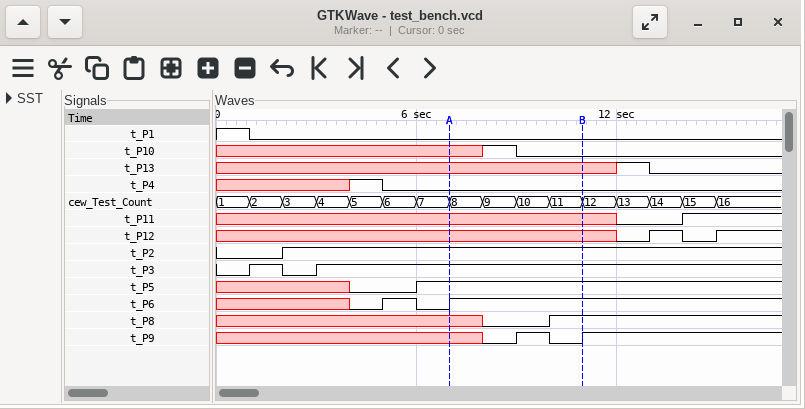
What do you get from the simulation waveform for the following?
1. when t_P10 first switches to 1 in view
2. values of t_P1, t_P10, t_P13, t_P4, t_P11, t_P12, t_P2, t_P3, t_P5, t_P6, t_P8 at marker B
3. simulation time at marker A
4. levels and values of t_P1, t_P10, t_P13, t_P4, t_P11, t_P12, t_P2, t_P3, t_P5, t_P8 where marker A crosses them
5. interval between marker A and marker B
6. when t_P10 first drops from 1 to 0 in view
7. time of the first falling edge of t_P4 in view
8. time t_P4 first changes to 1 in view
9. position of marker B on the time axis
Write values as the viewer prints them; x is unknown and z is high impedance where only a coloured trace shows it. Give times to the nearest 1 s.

8 s
t_P1=0, t_P10=0, t_P13=x, t_P4=0, t_P11=x, t_P12=x, t_P2=1, t_P3=1, t_P5=1, t_P6=1, t_P8=1
7 s
t_P1=0, t_P10=x, t_P13=x, t_P4=0, t_P11=x, t_P12=x, t_P2=1, t_P3=1, t_P5=1, t_P8=x
4 s
9 s
5 s
4 s
11 s
